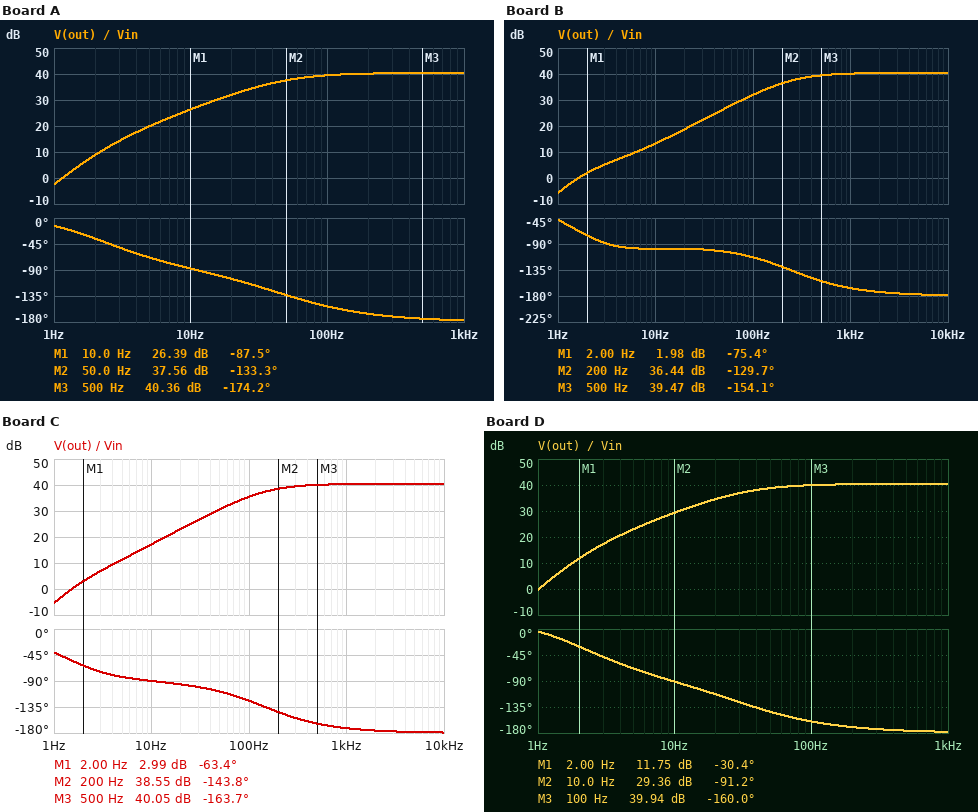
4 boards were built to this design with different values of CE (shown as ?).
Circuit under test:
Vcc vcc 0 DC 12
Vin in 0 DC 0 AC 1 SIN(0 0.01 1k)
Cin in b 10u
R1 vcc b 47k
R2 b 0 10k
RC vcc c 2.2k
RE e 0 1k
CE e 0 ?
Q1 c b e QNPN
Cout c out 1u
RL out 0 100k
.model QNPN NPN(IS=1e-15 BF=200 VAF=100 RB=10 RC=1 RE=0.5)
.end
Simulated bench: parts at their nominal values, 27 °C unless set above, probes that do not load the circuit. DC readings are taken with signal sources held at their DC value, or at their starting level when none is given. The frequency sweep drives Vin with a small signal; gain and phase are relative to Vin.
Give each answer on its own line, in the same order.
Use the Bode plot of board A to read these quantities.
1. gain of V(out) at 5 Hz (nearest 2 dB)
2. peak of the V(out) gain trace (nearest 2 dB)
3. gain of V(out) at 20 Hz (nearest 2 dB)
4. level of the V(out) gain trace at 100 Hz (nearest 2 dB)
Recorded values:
20 dB
40 dB
32 dB
40 dB
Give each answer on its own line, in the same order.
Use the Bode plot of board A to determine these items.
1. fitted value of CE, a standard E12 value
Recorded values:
180 µF
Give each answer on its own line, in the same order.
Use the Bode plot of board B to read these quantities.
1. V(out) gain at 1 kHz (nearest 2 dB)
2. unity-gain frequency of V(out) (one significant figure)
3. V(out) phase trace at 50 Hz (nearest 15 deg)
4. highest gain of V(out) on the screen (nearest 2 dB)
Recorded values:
40 dB
2 Hz
-105 deg
40 dB
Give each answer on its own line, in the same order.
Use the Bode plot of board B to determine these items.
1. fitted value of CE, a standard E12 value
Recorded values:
33 µF
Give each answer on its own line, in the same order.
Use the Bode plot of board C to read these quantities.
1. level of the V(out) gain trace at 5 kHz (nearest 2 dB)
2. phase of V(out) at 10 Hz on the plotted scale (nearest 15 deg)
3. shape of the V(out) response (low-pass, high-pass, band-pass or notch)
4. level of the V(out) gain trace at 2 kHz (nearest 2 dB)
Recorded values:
40 dB
-90 deg
high-pass
40 dB
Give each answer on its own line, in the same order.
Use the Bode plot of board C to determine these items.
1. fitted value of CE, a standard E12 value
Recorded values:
56 µF
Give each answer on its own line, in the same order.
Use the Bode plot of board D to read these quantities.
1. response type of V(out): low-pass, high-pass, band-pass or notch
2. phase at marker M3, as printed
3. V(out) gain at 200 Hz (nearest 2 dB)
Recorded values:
high-pass
-160.0 deg
40 dB
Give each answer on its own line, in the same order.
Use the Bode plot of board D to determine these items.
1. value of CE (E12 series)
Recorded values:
270 µF
